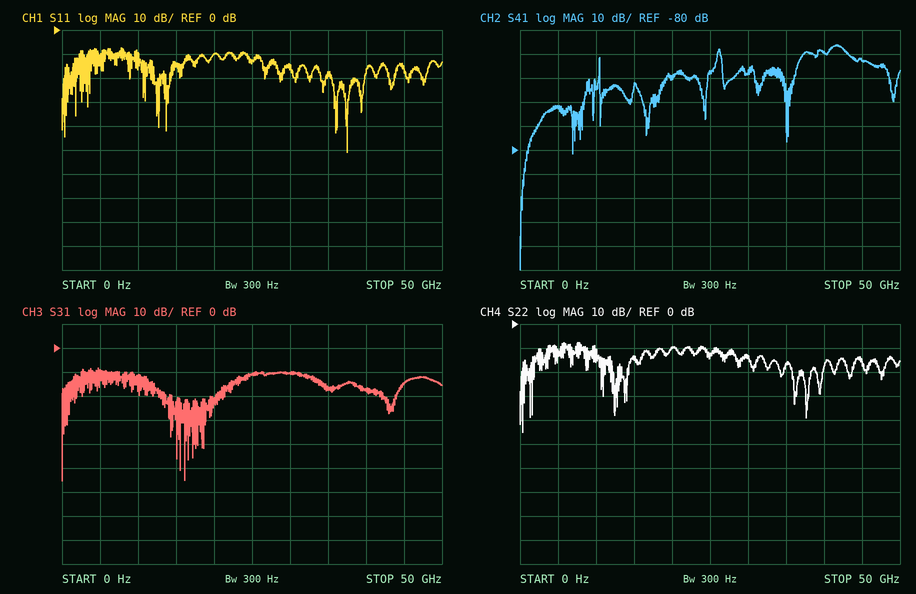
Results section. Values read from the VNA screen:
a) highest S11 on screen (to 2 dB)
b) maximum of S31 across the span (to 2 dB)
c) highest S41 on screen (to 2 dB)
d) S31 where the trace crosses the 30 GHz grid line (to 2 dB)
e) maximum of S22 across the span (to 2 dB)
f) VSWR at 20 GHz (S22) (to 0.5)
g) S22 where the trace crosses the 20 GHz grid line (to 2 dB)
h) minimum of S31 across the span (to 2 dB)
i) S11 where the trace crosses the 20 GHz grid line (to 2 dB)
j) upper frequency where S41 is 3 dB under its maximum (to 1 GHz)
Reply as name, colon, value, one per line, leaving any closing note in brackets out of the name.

highest S11 on screen: -8 dB
maximum of S31 across the span: -8 dB
highest S41 on screen: -36 dB
S31 where the trace crosses the 30 GHz grid line: -10 dB
maximum of S22 across the span: -8 dB
VSWR at 20 GHz (S22): 2.0
S22 where the trace crosses the 20 GHz grid line: -10 dB
minimum of S31 across the span: -56 dB
S11 where the trace crosses the 20 GHz grid line: -10 dB
upper frequency where S41 is 3 dB under its maximum: 43 GHz
